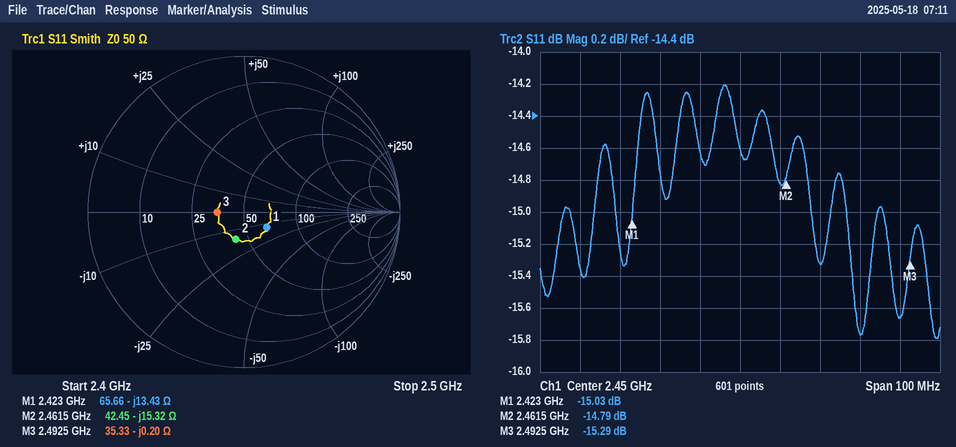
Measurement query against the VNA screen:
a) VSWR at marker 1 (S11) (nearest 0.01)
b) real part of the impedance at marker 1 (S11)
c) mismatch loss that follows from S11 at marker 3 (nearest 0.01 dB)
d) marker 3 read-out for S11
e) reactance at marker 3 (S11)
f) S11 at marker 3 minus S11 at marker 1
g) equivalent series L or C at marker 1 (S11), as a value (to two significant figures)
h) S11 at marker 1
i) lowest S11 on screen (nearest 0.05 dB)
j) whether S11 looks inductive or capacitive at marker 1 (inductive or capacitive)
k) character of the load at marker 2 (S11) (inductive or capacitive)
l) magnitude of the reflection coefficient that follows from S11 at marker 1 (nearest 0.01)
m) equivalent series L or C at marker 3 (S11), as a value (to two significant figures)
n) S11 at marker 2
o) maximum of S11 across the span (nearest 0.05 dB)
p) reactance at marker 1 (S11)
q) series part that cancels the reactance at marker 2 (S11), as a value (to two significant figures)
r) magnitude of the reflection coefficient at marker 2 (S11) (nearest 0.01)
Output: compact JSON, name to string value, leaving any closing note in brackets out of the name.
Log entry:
{"VSWR at marker 1 (S11)": "1.43", "real part of the impedance at marker 1": "65.66 Ω", "mismatch loss that follows from S11 at marker 3": "0.13 dB", "marker 3 read-out for S11": "-15.29 dB", "reactance at marker 3": "-0.20 Ω", "S11 at marker 3 minus S11 at marker 1": "-0.26 dB", "equivalent series L or C at marker 1 (S11), as a value": "4.9 pF", "S11 at marker 1": "-15.03 dB", "lowest S11 on screen": "-15.80 dB", "whether S11 looks inductive or capacitive at marker 1": "capacitive", "character of the load at marker 2 (S11)": "capacitive", "magnitude of the reflection coefficient that follows from S11 at marker 1": "0.18", "equivalent series L or C at marker 3 (S11), as a value": "320 pF", "S11 at marker 2": "-14.79 dB", "maximum of S11 across the span": "-14.20 dB", "reactance at marker 1": "-13.43 Ω", "series part that cancels the reactance at marker 2 (S11), as a value": "990 pH", "magnitude of the reflection coefficient at marker 2 (S11)": "0.18"}
